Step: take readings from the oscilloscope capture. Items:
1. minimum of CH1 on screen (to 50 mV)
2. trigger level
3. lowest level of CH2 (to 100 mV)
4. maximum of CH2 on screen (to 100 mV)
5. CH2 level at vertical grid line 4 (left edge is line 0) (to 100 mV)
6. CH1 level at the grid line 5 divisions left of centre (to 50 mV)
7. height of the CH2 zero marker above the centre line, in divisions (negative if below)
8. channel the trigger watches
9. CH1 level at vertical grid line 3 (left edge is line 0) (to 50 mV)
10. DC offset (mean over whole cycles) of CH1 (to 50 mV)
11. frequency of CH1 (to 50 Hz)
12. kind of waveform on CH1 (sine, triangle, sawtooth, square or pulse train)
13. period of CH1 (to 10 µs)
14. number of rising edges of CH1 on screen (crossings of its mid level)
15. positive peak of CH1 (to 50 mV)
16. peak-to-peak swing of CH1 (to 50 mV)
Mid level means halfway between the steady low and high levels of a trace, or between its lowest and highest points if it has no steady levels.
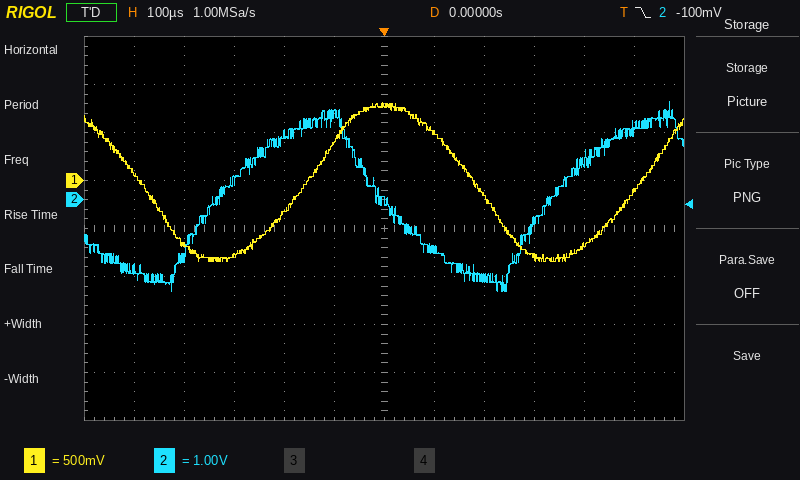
-850 mV
-100 mV
-1.9 V
2.0 V
1.4 V
100 mV
+0.6 div
CH2
-800 mV
0 mV
1.50 kHz
sine
670 µs
2
800 mV
1.65 V
